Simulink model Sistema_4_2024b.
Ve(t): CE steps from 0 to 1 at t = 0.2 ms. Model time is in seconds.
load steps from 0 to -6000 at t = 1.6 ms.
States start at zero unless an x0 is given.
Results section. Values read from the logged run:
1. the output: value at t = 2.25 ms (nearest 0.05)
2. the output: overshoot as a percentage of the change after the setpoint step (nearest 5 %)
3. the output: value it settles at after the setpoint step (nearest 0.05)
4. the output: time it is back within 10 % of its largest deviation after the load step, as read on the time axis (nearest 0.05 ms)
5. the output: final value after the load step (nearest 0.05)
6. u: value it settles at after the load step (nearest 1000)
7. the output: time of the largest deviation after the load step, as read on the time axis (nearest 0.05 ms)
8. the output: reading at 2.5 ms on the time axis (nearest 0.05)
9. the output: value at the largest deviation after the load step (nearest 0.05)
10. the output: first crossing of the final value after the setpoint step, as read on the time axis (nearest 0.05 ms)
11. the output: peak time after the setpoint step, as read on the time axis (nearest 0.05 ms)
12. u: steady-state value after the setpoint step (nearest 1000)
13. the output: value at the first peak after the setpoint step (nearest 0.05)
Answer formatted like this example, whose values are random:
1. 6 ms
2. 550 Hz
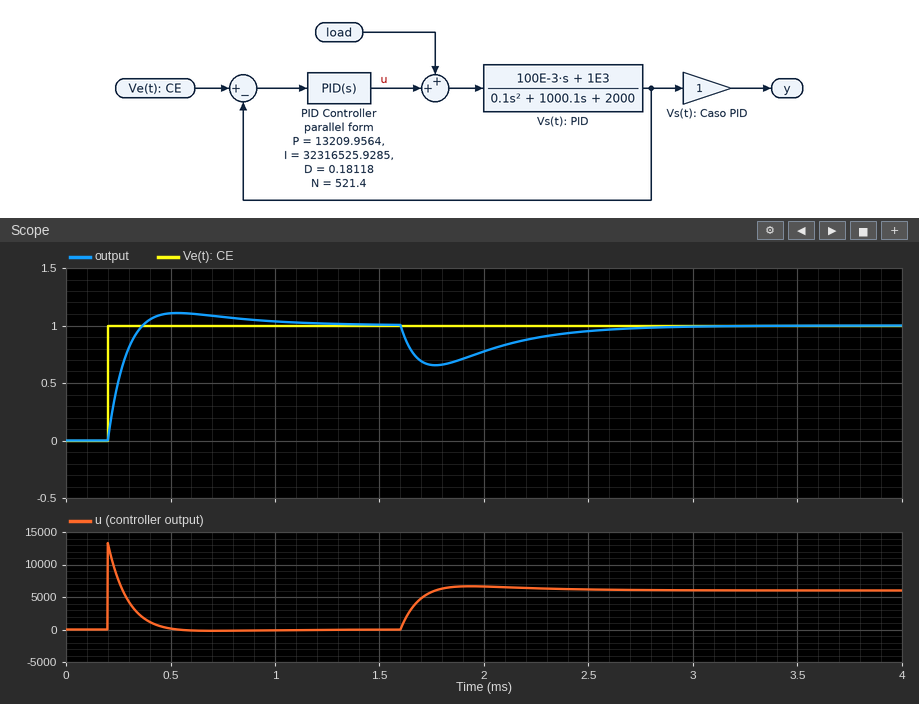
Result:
1. 0.90
2. 10 %
3. 1.00
4. 2.60 ms
5. 1.00
6. 6000
7. 1.75 ms
8. 0.95
9. 0.65
10. 0.35 ms
11. 0.55 ms
12. 0
13. 1.10
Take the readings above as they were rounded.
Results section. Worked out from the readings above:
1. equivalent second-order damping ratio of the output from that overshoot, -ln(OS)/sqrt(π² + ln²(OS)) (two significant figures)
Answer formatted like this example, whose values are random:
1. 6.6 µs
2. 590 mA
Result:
1. 0.59
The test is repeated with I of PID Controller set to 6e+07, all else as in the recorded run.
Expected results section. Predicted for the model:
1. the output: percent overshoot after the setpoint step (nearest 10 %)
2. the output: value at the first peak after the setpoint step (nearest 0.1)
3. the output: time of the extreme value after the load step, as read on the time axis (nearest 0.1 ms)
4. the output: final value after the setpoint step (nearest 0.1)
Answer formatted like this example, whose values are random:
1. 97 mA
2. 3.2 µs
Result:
1. 20 %
2. 1.2
3. 1.7 ms
4. 1.0
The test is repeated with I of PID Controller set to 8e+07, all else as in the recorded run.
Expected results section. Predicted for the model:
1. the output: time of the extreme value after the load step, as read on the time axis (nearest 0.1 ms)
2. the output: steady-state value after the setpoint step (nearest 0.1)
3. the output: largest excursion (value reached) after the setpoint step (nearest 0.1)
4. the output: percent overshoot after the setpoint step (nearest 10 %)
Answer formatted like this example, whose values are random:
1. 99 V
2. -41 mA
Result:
1. 1.7 ms
2. 1.0
3. 1.2
4. 20 %
